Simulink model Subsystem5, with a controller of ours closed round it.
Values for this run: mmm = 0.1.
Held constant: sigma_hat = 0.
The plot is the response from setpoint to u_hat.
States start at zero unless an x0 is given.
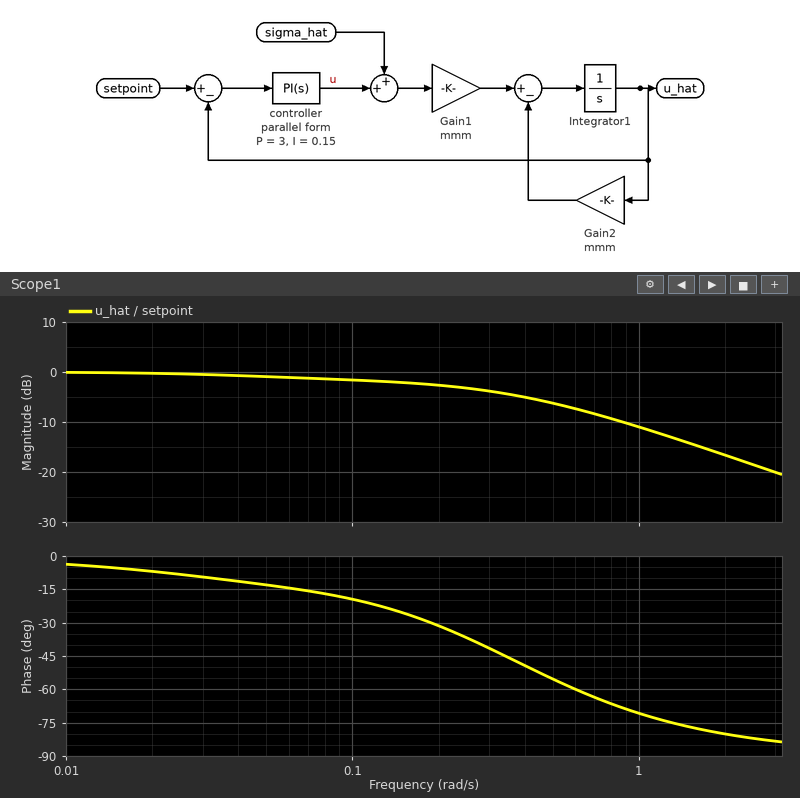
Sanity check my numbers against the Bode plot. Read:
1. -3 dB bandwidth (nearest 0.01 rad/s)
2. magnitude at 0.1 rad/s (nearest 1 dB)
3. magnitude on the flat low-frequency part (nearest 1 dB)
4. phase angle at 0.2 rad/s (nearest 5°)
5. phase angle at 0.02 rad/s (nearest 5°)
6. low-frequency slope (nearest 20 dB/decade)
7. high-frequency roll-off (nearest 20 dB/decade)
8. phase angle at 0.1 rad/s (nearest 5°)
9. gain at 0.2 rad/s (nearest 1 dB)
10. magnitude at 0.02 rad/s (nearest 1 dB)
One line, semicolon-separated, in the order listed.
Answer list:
0.24 rad/s; -2 dB; 0 dB; -30°; -5°; 0 dB/decade; -20 dB/decade; -20°; -3 dB; 0 dB
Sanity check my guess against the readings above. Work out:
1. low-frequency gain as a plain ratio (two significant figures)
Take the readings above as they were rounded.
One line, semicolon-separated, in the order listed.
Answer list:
1.0
